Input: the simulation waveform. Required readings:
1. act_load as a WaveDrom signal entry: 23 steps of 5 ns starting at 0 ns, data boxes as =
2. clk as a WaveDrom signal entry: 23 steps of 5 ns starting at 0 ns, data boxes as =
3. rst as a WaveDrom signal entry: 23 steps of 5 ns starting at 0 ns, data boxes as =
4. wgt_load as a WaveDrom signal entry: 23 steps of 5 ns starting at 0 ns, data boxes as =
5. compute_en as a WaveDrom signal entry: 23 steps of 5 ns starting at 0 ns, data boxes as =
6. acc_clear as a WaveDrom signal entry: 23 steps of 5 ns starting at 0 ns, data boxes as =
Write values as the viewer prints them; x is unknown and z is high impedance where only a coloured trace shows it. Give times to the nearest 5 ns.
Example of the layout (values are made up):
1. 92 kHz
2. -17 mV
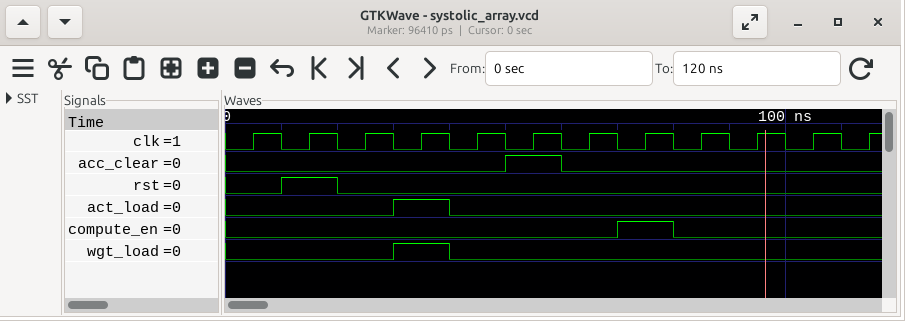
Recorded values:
1. {name: 'act_load', wave: '0.....1.0..............'}
2. {name: 'clk', wave: '01010101010101010101010'}
3. {name: 'rst', wave: '0.1.0..................'}
4. {name: 'wgt_load', wave: '0.....1.0..............'}
5. {name: 'compute_en', wave: '0.............1.0......'}
6. {name: 'acc_clear', wave: '0.........1.0..........'}
